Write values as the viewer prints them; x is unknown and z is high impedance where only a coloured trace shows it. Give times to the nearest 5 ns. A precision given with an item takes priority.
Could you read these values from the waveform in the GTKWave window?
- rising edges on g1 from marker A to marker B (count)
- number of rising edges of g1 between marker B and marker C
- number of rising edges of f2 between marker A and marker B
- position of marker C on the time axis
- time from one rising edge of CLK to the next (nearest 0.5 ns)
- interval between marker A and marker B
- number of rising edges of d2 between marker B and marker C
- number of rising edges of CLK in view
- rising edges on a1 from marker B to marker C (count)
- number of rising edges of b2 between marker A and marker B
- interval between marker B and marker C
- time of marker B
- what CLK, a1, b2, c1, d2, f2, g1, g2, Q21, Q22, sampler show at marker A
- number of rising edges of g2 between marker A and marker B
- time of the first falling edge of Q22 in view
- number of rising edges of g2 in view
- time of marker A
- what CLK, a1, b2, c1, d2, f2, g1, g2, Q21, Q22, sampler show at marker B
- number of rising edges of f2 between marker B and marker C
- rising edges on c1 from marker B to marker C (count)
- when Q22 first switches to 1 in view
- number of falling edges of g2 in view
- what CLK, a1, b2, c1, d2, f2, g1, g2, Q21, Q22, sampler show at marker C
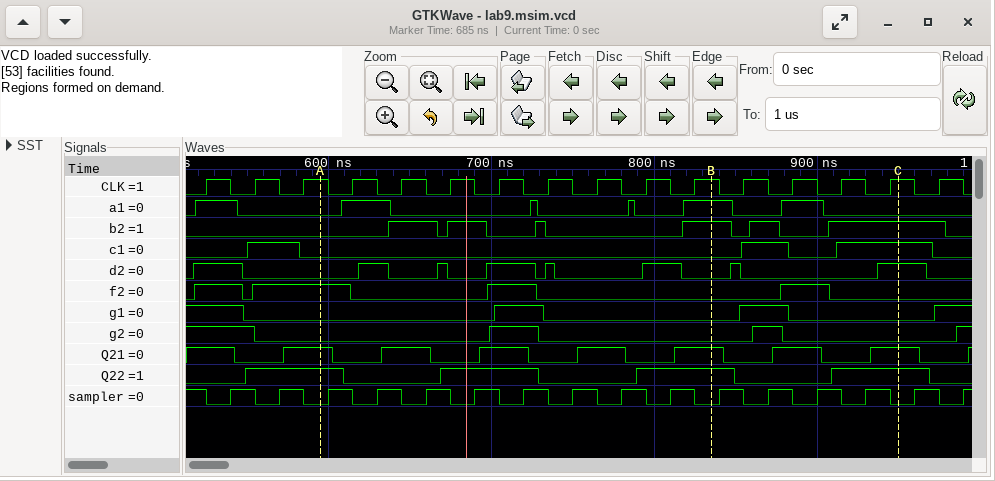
1
1
1
950 ns
30 ns
240 ns
2
16
1
4
115 ns
835 ns
CLK=1, a1=0, b2=0, c1=0, d2=0, f2=1, g1=0, g2=0, Q21=1, Q22=1, sampler=0
1
610 ns
3
595 ns
CLK=1, a1=1, b2=1, c1=0, d2=0, f2=0, g1=0, g2=0, Q21=1, Q22=1, sampler=0
1
2
550 ns
3
CLK=1, a1=0, b2=1, c1=1, d2=1, f2=0, g1=0, g2=0, Q21=1, Q22=1, sampler=0
